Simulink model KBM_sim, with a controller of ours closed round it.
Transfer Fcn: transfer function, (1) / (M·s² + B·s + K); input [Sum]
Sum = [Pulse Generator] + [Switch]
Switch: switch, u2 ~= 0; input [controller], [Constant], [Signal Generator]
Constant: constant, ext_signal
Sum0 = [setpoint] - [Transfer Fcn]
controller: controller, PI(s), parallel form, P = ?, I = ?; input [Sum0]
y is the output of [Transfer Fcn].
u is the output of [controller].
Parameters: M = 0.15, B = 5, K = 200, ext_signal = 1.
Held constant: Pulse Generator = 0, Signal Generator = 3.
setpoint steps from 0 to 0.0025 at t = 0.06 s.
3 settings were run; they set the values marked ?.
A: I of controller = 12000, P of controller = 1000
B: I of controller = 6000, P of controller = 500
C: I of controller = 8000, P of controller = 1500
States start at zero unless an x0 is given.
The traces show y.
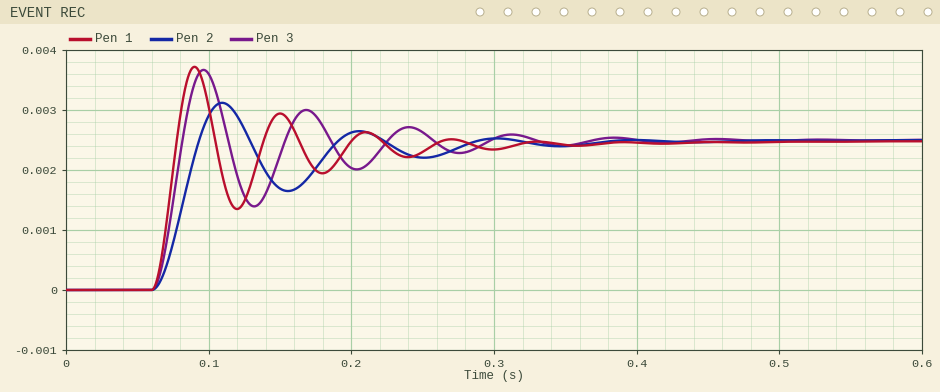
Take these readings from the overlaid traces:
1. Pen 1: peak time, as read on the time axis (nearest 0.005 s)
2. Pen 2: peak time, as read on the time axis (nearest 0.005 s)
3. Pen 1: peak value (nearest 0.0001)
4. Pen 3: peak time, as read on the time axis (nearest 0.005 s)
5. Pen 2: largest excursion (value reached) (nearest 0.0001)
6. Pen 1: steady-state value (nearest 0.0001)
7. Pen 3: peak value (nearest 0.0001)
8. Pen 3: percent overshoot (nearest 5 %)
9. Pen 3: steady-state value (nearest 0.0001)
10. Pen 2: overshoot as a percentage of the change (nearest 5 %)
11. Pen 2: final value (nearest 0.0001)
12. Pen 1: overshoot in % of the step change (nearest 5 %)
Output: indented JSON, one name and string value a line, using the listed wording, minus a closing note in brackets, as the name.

{
  "Pen 1: peak time, as read on the time axis": "0.090 s",
  "Pen 2: peak time, as read on the time axis": "0.110 s",
  "Pen 1: peak value": "0.0037",
  "Pen 3: peak time, as read on the time axis": "0.095 s",
  "Pen 2: largest excursion (value reached)": "0.0031",
  "Pen 1: steady-state value": "0.0025",
  "Pen 3: peak value": "0.0037",
  "Pen 3: percent overshoot": "45 %",
  "Pen 3: steady-state value": "0.0025",
  "Pen 2: overshoot as a percentage of the change": "25 %",
  "Pen 2: final value": "0.0025",
  "Pen 1: overshoot in % of the step change": "50 %"
}
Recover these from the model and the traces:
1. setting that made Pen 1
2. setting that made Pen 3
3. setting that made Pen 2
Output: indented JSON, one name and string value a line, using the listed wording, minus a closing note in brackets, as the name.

{
  "setting that made Pen 1": "C",
  "setting that made Pen 3": "A",
  "setting that made Pen 2": "B"
}
